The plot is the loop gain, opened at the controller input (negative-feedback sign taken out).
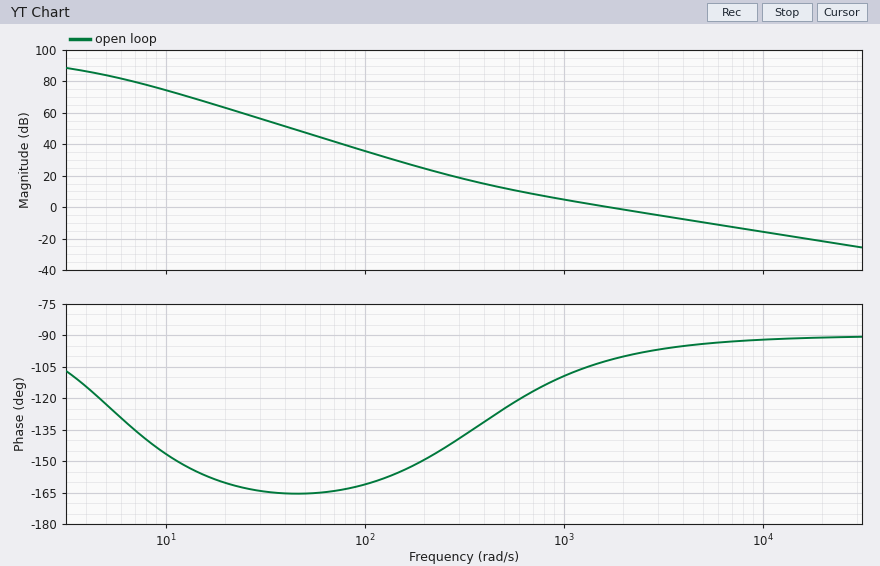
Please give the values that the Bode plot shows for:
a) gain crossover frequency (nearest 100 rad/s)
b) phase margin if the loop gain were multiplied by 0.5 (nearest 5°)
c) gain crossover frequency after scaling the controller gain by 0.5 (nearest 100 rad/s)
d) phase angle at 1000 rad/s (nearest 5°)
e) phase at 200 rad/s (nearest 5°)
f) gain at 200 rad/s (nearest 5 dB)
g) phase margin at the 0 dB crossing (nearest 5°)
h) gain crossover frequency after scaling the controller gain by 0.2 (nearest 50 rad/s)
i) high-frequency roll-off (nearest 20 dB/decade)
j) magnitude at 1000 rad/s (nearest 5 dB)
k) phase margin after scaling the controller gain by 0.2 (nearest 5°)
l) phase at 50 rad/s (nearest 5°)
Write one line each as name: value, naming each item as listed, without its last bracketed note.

gain crossover frequency: 1700 rad/s
phase margin if the loop gain were multiplied by 0.5: 70°
gain crossover frequency after scaling the controller gain by 0.5: 900 rad/s
phase angle at 1000 rad/s: -110°
phase at 200 rad/s: -150°
gain at 200 rad/s: 25 dB
phase margin at the 0 dB crossing: 80°
gain crossover frequency after scaling the controller gain by 0.2: 450 rad/s
high-frequency roll-off: -20 dB/decade
magnitude at 1000 rad/s: 5 dB
phase margin after scaling the controller gain by 0.2: 50°
phase at 50 rad/s: -165°
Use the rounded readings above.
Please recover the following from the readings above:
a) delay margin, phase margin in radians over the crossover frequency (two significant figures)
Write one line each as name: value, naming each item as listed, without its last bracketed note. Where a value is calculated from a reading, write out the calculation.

delay margin, phase margin in radians over the crossover frequency: 80 × π / 180 / 1700 = 0.00082 s
